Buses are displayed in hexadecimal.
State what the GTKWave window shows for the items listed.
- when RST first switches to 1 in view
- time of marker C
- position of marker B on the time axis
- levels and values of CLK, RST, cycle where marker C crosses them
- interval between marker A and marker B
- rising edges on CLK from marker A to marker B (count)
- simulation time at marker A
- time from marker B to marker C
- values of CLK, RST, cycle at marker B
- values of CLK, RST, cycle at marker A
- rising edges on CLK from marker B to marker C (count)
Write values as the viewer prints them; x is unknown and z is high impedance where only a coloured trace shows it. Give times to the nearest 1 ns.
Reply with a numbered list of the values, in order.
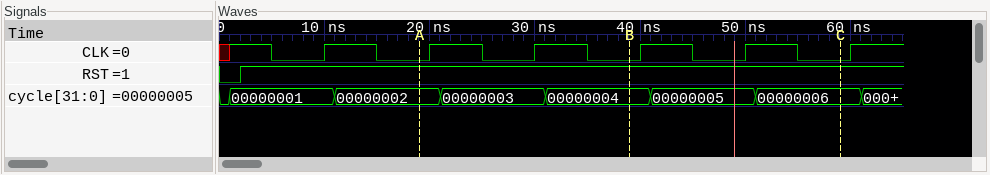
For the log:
1. 2 ns
2. 59 ns
3. 39 ns
4. CLK=0, RST=1, cycle=00000006
5. 20 ns
6. 2
7. 19 ns
8. 20 ns
9. CLK=0, RST=1, cycle=00000004
10. CLK=0, RST=1, cycle=00000002
11. 2
